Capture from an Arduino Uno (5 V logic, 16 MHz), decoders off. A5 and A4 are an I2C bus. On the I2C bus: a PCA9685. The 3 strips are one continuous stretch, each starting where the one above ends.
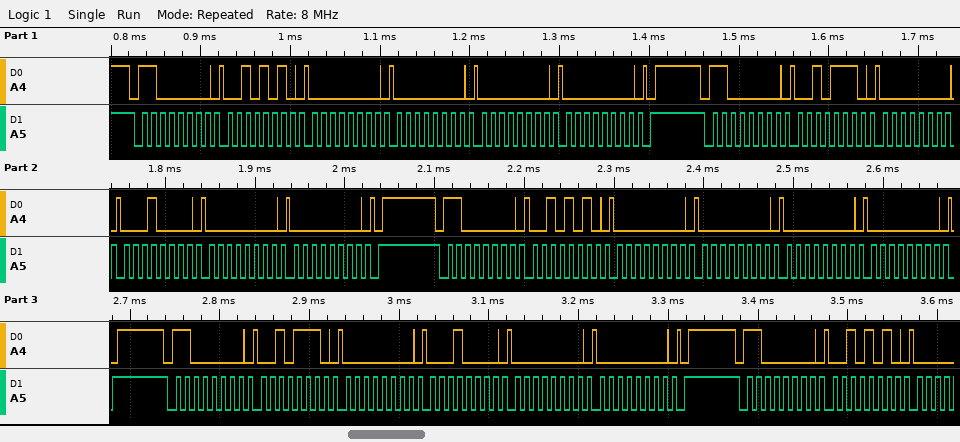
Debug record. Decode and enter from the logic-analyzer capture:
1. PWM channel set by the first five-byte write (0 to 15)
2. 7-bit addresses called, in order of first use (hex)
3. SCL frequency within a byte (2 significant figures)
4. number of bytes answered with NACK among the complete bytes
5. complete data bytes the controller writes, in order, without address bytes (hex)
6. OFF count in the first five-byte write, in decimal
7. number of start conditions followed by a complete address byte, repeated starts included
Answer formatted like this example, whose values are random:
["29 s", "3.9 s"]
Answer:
["9", "0x60", "100 kHz", "0", "2A 00 00 00 00 2E 00 10 00 00 2A 00 00 00 00 2E 00 10 00 00 2A", "0", "5"]
